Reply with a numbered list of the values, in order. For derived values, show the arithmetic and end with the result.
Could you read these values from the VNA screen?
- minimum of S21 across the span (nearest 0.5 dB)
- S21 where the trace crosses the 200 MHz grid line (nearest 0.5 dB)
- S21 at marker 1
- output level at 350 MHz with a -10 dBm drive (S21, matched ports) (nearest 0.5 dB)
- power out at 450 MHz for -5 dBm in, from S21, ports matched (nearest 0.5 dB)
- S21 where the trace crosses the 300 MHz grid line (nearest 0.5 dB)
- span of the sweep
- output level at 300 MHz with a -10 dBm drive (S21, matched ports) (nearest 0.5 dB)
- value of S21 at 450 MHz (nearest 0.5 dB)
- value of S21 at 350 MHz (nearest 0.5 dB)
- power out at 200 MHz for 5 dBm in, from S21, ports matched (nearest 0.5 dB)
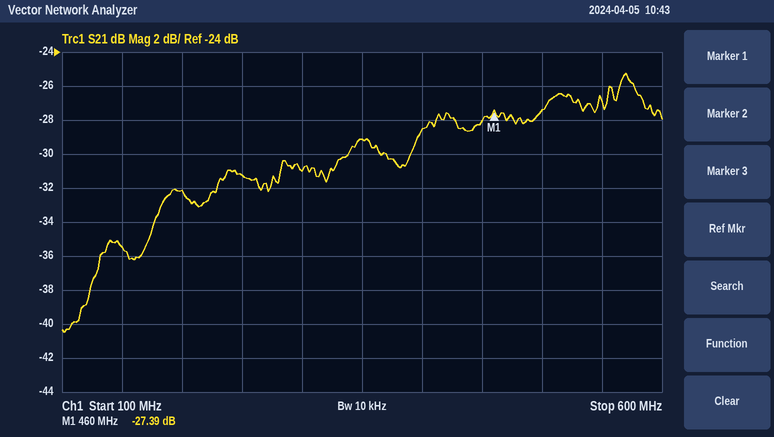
1. -40.5 dB
2. -32.0 dB
3. -27.39 dB
4. -10 dBm + (-29.0 dB) = -39.0 dBm
5. -5 dBm + (-28.0 dB) = -33.0 dBm
6. -31.0 dB
7. 500 MHz
8. -10 dBm + (-31.0 dB) = -41.0 dBm
9. -28.0 dB
10. -29.0 dB
11. 5 dBm + (-32.0 dB) = -27.0 dBm
